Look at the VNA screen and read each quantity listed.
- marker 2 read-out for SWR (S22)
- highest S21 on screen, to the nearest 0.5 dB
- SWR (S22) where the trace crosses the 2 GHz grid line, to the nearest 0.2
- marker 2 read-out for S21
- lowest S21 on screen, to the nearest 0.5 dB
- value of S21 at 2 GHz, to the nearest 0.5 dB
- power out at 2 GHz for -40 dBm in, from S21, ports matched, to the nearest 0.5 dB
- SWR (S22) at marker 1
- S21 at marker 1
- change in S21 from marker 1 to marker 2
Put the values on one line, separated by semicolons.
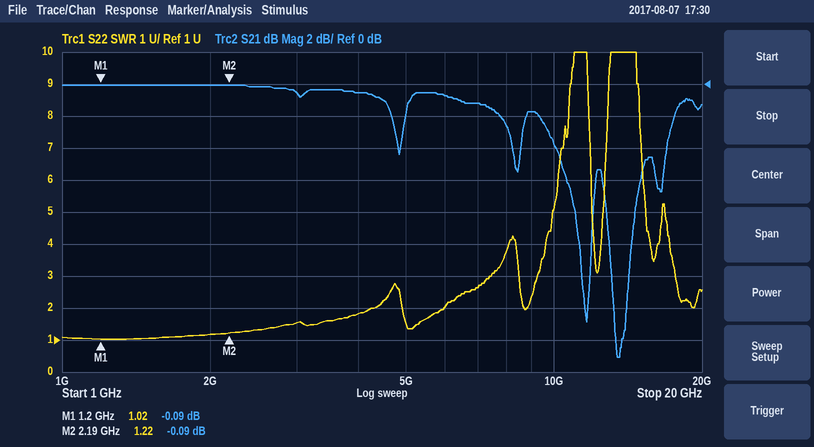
1.22; 0.0 dB; 1.2; -0.09 dB; -17.0 dB; 0.0 dB; -40.0 dBm; 1.02; -0.09 dB; 0.00 dB
